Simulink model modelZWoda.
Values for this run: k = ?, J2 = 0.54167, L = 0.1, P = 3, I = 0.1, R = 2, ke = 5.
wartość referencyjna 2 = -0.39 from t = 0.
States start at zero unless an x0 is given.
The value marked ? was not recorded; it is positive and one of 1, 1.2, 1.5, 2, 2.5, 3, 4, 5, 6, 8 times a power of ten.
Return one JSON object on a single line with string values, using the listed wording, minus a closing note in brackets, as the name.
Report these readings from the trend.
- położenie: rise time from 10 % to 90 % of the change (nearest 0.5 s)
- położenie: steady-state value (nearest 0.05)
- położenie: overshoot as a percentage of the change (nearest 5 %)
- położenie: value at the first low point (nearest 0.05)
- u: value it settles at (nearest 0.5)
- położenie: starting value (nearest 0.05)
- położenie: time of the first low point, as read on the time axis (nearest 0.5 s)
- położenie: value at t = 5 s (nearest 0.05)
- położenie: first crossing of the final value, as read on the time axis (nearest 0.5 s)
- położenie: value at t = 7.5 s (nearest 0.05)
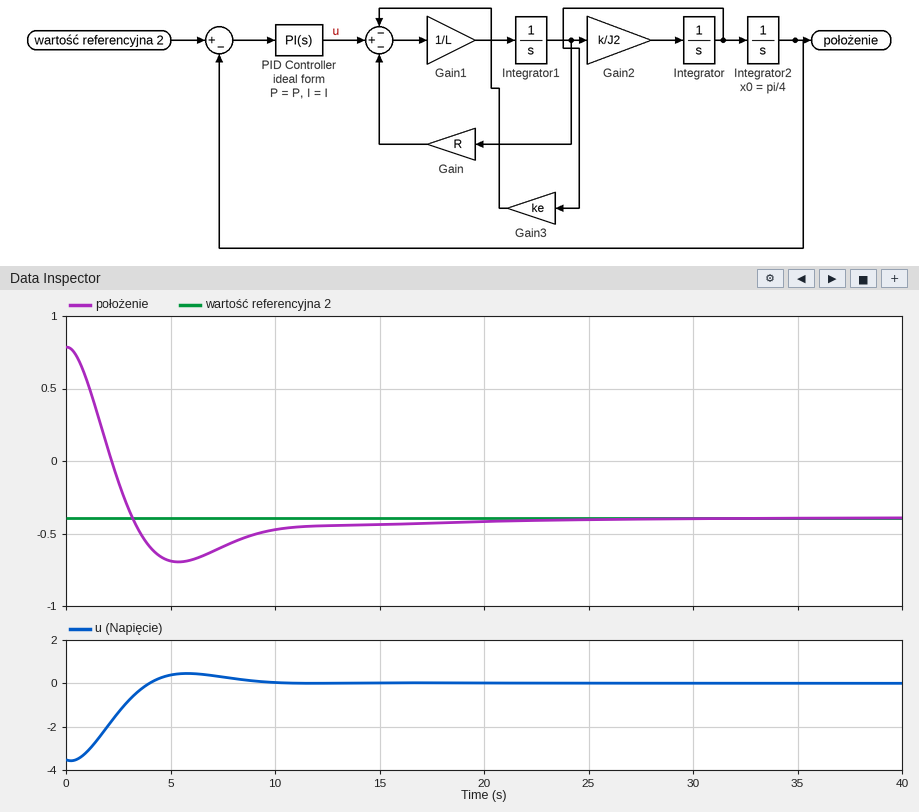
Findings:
{"położenie: rise time from 10 % to 90 % of the change": "2.0 s", "położenie: steady-state value": "-0.40", "położenie: overshoot as a percentage of the change": "25 %", "położenie: value at the first low point": "-0.70", "u: value it settles at": "0.0", "położenie: starting value": "0.80", "położenie: time of the first low point, as read on the time axis": "5.5 s", "położenie: value at t = 5 s": "-0.70", "położenie: first crossing of the final value, as read on the time axis": "3.0 s", "położenie: value at t = 7.5 s": "-0.60"}
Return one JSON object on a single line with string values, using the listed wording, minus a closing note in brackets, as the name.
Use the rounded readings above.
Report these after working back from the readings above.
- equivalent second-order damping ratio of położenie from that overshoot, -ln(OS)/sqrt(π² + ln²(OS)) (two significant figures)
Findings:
{"equivalent second-order damping ratio of położenie from that overshoot, -ln(OS)/sqrt(π² + ln²(OS))": "0.40"}
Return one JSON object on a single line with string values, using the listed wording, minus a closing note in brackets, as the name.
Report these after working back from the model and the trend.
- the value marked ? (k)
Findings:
{"the value marked ?": "0.2"}
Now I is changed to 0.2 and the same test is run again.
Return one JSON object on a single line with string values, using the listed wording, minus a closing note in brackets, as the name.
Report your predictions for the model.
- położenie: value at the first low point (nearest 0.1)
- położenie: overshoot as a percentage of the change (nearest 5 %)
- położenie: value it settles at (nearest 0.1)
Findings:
{"położenie: value at the first low point": "-0.9", "położenie: overshoot as a percentage of the change": "40 %", "położenie: value it settles at": "-0.4"}
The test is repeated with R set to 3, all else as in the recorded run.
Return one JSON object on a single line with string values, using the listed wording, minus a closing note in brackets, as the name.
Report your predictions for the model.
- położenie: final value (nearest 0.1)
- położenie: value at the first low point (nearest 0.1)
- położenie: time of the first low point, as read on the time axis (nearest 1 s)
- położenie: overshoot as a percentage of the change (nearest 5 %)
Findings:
{"położenie: final value": "-0.4", "położenie: value at the first low point": "-0.8", "położenie: time of the first low point, as read on the time axis": "6 s", "położenie: overshoot as a percentage of the change": "35 %"}
